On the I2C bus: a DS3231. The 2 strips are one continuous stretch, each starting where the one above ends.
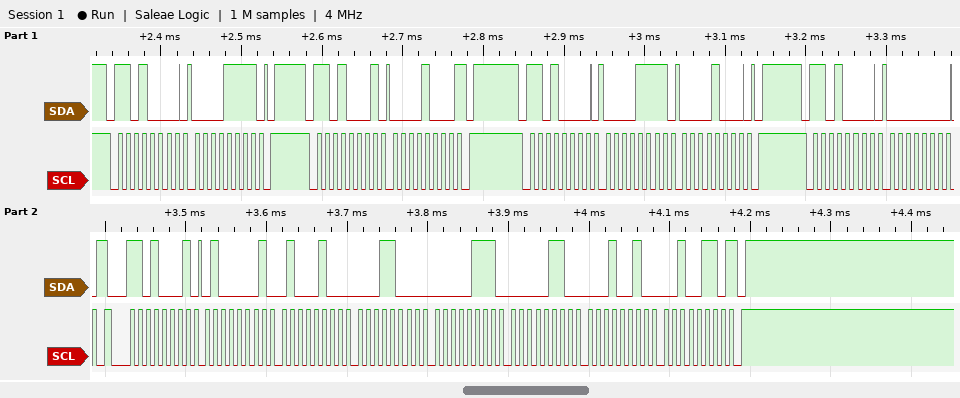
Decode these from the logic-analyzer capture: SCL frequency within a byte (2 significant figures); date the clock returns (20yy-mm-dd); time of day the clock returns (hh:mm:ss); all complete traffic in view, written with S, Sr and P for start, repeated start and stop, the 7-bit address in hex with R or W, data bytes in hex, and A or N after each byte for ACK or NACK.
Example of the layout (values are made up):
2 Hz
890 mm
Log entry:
100 kHz
2026-12-06
18:44:41
S 68W A 0F A P S 68R A 08 N P S 68W A 0F A 08 A P S 68W A 00 A Sr 68R A 41 A 44 A 18 A 07 A 06 A 12 A 26 N P
